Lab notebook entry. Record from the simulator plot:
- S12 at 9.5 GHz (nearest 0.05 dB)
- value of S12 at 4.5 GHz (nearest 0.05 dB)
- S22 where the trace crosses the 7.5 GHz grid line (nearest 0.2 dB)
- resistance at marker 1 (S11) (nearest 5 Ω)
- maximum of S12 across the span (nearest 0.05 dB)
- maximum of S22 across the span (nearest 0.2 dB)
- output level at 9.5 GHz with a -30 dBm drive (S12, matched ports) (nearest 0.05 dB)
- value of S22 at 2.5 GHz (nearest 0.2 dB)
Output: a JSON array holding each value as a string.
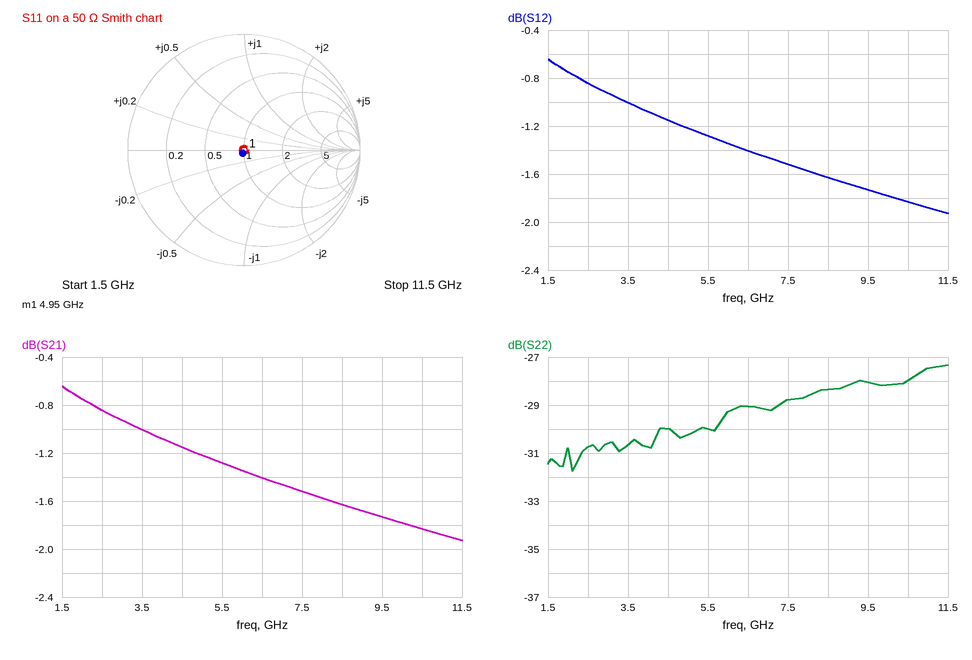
["-1.75 dB", "-1.15 dB", "-28.8 dB", "50 Ω", "-0.65 dB", "-27.4 dB", "-31.75 dBm", "-30.8 dB"]
